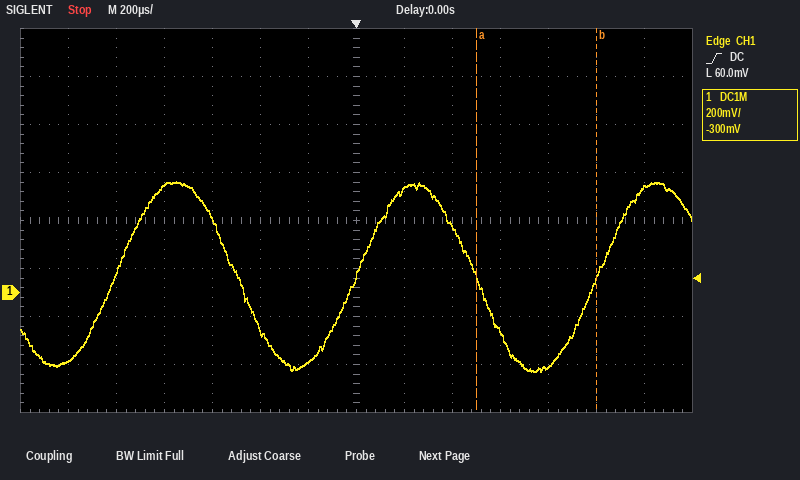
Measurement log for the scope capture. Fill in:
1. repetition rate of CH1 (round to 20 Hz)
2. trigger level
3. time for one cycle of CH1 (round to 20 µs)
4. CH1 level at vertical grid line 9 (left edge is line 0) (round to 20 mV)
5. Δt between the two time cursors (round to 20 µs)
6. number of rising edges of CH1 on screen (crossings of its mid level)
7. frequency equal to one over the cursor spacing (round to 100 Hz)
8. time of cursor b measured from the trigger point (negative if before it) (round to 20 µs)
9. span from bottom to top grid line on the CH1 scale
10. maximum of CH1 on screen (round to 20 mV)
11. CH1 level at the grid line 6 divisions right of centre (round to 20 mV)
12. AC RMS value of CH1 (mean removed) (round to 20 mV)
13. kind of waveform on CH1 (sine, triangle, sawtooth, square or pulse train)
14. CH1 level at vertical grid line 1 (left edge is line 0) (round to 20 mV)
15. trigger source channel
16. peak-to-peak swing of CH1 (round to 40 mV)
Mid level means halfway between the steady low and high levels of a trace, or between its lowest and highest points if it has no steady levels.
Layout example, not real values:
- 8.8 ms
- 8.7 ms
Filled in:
- 1.00 kHz
- 60.0 mV
- 1.00 ms
- 280 mV
- 500 µs
- 3
- 2.0 kHz
- +1.00 ms
- 1.6 V
- 460 mV
- 440 mV
- 280 mV
- sine
- -280 mV
- CH1
- 800 mV
